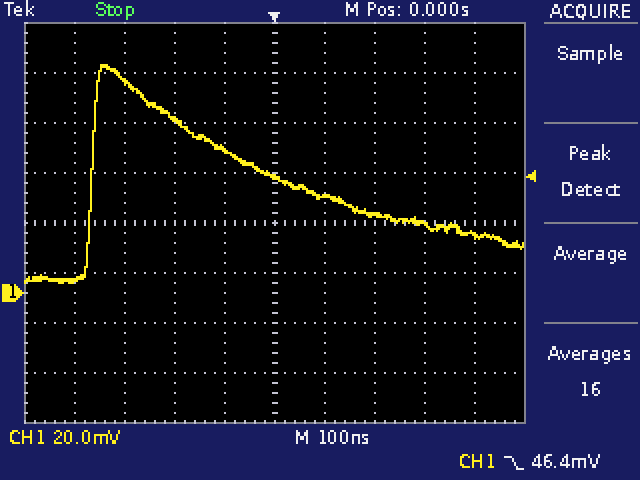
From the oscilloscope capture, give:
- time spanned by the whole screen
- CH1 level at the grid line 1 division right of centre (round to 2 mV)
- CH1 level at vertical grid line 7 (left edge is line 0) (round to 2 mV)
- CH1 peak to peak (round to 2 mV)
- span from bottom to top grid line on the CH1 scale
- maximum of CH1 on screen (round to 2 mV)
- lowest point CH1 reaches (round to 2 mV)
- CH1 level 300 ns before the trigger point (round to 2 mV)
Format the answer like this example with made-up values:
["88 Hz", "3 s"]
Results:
["1 µs", "38 mV", "32 mV", "88 mV", "160 mV", "92 mV", "4 mV", "84 mV"]
